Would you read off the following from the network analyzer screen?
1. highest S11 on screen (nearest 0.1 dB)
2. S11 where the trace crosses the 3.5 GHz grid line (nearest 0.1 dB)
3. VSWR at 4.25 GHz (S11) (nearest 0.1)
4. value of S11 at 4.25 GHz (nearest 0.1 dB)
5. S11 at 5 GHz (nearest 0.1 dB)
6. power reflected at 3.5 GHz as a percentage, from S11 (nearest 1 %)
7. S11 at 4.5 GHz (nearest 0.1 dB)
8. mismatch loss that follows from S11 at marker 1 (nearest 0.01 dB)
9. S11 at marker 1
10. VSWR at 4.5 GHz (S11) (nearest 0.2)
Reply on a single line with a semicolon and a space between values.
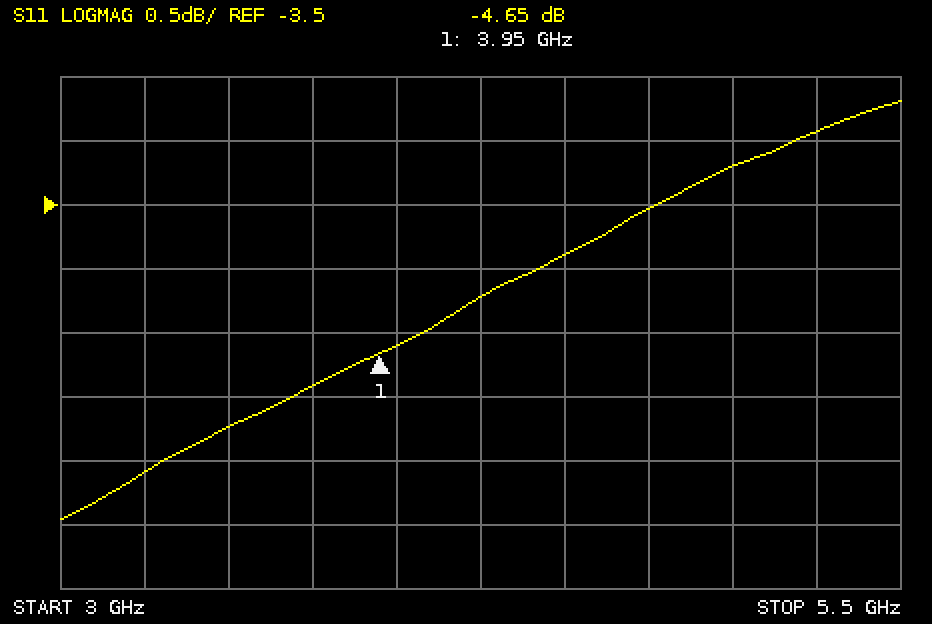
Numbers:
-2.7 dB; -5.2 dB; 4.2; -4.2 dB; -3.2 dB; 30 %; -3.9 dB; 1.82 dB; -4.65 dB; 4.6
